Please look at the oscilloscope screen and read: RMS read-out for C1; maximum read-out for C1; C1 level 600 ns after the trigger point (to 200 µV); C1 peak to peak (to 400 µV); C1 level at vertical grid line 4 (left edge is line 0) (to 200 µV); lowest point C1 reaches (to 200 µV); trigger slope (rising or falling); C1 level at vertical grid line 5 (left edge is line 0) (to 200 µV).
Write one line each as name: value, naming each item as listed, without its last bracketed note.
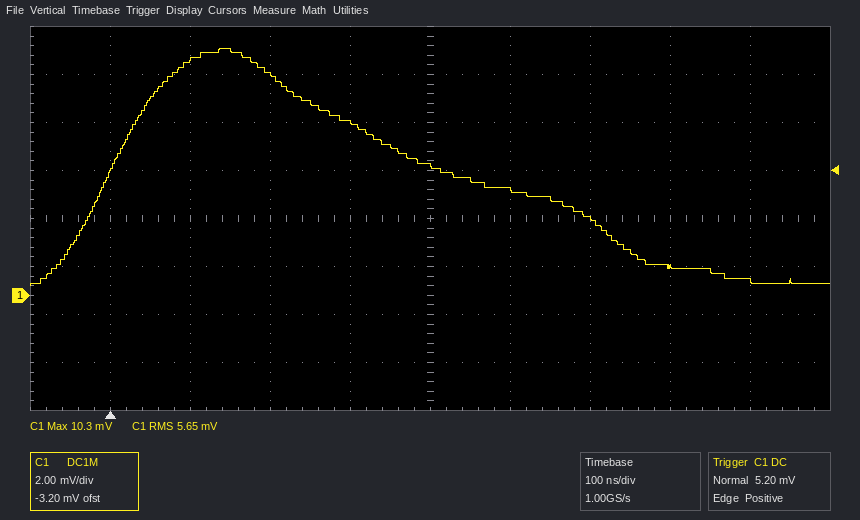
RMS read-out for C1: 5.65 mV
maximum read-out for C1: 10.3 mV
C1 level 600 ns after the trigger point: 3.2 mV
C1 peak to peak: 10.0 mV
C1 level at vertical grid line 4 (left edge is line 0): 7.2 mV
lowest point C1 reaches: 400 µV
trigger slope: rising
C1 level at vertical grid line 5 (left edge is line 0): 5.4 mV
